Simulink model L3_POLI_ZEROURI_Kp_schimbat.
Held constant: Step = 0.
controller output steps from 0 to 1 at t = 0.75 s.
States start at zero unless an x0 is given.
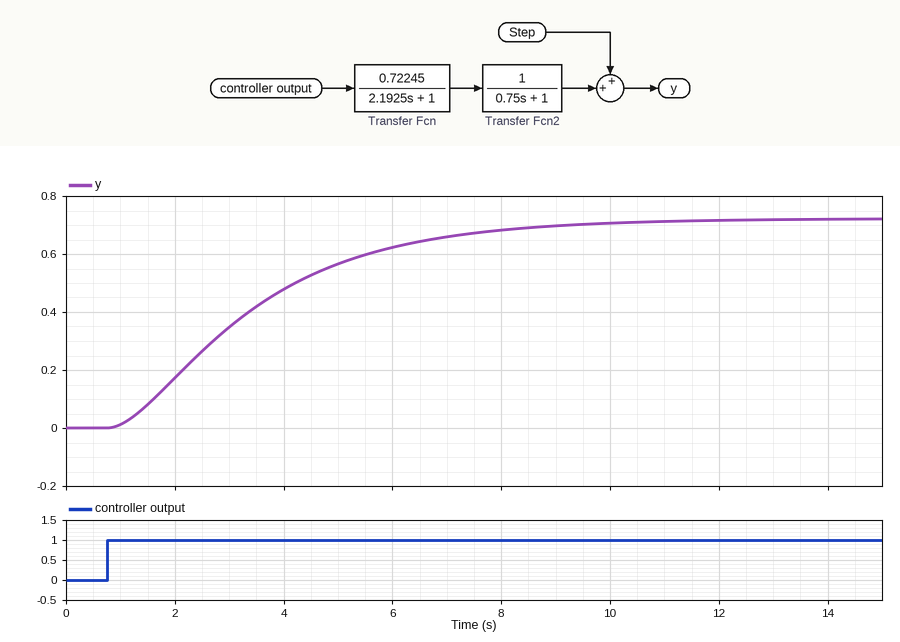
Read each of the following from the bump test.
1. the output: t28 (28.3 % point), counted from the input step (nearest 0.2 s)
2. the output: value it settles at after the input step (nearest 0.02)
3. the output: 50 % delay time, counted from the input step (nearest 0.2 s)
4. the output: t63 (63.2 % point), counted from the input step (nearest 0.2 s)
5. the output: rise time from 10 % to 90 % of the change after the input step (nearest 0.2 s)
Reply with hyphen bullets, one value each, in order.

- 1.4 s
- 0.72
- 2.4 s
- 3.0 s
- 5.2 s
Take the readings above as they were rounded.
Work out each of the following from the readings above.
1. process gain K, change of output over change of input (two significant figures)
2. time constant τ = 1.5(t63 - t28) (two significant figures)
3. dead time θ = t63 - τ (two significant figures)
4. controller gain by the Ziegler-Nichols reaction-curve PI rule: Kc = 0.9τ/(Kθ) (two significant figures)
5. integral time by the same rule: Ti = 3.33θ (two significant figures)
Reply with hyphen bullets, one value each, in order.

- 0.72
- 2.4 s
- 0.60 s
- 5.0
- 2.0 s
